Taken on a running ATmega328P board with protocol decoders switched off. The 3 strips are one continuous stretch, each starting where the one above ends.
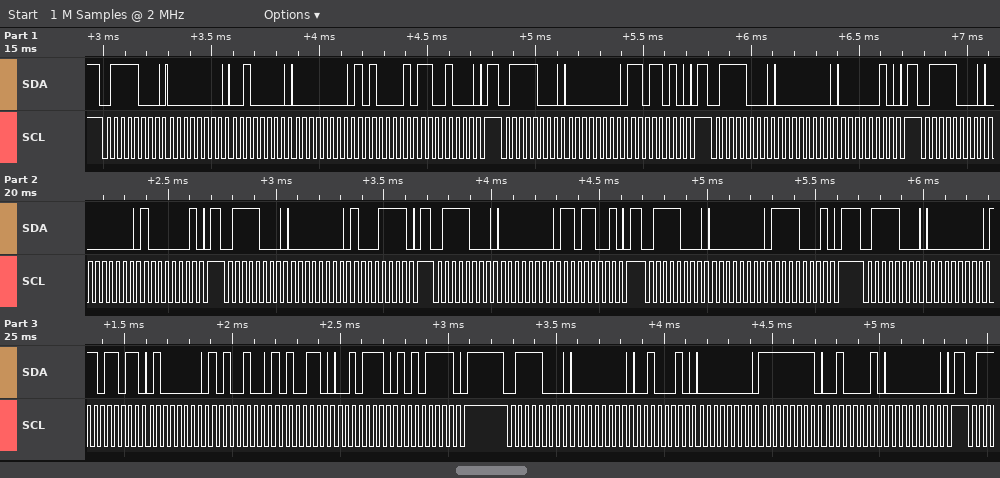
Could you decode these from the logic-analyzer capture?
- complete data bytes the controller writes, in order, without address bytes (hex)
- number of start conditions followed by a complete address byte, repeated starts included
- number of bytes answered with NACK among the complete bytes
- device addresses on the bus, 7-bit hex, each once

00 20 00 A1 C8 00 DA 00 02 00 81 00 8F 00 D9 00 F1 00 DB 40 A4 A6 2E AF 00 22 00 FF 21 00
9
0
0x3C
